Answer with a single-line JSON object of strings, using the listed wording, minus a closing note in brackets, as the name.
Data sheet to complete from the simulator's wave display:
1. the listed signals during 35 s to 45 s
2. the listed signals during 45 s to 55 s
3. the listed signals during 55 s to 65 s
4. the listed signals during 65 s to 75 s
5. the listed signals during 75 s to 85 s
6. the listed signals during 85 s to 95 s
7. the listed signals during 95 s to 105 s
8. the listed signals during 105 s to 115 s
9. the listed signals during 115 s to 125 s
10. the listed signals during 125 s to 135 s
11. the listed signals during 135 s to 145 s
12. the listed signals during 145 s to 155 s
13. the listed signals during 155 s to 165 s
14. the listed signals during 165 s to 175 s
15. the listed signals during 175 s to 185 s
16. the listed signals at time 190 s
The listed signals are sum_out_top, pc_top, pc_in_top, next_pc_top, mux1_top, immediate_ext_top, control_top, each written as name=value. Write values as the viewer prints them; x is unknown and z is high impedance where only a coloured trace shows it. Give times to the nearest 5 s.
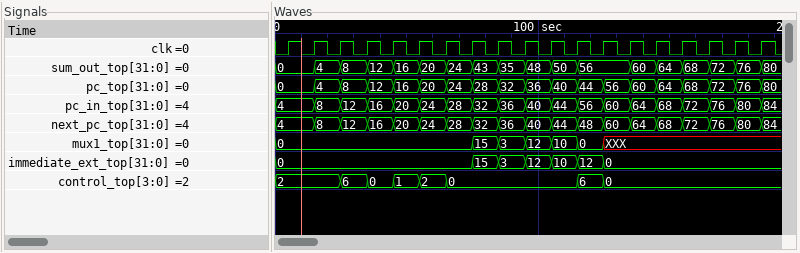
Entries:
{"the listed signals during 35 s to 45 s": "sum_out_top=12, pc_top=12, pc_in_top=16, next_pc_top=16, mux1_top=0, immediate_ext_top=0, control_top=0", "the listed signals during 45 s to 55 s": "sum_out_top=16, pc_top=16, pc_in_top=20, next_pc_top=20, mux1_top=0, immediate_ext_top=0, control_top=1", "the listed signals during 55 s to 65 s": "sum_out_top=20, pc_top=20, pc_in_top=24, next_pc_top=24, mux1_top=0, immediate_ext_top=0, control_top=2", "the listed signals during 65 s to 75 s": "sum_out_top=24, pc_top=24, pc_in_top=28, next_pc_top=28, mux1_top=0, immediate_ext_top=0, control_top=0", "the listed signals during 75 s to 85 s": "sum_out_top=43, pc_top=28, pc_in_top=32, next_pc_top=32, mux1_top=15, immediate_ext_top=15, control_top=0", "the listed signals during 85 s to 95 s": "sum_out_top=35, pc_top=32, pc_in_top=36, next_pc_top=36, mux1_top=3, immediate_ext_top=3, control_top=0", "the listed signals during 95 s to 105 s": "sum_out_top=48, pc_top=36, pc_in_top=40, next_pc_top=40, mux1_top=12, immediate_ext_top=12, control_top=0", "the listed signals during 105 s to 115 s": "sum_out_top=50, pc_top=40, pc_in_top=44, next_pc_top=44, mux1_top=10, immediate_ext_top=10, control_top=0", "the listed signals during 115 s to 125 s": "sum_out_top=56, pc_top=44, pc_in_top=56, next_pc_top=48, mux1_top=0, immediate_ext_top=12, control_top=6", "the listed signals during 125 s to 135 s": "sum_out_top=56, pc_top=56, pc_in_top=60, next_pc_top=60, mux1_top=XXX, immediate_ext_top=0, control_top=0", "the listed signals during 135 s to 145 s": "sum_out_top=60, pc_top=60, pc_in_top=64, next_pc_top=64, mux1_top=XXX, immediate_ext_top=0, control_top=0", "the listed signals during 145 s to 155 s": "sum_out_top=64, pc_top=64, pc_in_top=68, next_pc_top=68, mux1_top=XXX, immediate_ext_top=0, control_top=0", "the listed signals during 155 s to 165 s": "sum_out_top=68, pc_top=68, pc_in_top=72, next_pc_top=72, mux1_top=XXX, immediate_ext_top=0, control_top=0", "the listed signals during 165 s to 175 s": "sum_out_top=72, pc_top=72, pc_in_top=76, next_pc_top=76, mux1_top=XXX, immediate_ext_top=0, control_top=0", "the listed signals during 175 s to 185 s": "sum_out_top=76, pc_top=76, pc_in_top=80, next_pc_top=80, mux1_top=XXX, immediate_ext_top=0, control_top=0", "the listed signals at time 190 s": "sum_out_top=80, pc_top=80, pc_in_top=84, next_pc_top=84, mux1_top=XXX, immediate_ext_top=0, control_top=0"}
